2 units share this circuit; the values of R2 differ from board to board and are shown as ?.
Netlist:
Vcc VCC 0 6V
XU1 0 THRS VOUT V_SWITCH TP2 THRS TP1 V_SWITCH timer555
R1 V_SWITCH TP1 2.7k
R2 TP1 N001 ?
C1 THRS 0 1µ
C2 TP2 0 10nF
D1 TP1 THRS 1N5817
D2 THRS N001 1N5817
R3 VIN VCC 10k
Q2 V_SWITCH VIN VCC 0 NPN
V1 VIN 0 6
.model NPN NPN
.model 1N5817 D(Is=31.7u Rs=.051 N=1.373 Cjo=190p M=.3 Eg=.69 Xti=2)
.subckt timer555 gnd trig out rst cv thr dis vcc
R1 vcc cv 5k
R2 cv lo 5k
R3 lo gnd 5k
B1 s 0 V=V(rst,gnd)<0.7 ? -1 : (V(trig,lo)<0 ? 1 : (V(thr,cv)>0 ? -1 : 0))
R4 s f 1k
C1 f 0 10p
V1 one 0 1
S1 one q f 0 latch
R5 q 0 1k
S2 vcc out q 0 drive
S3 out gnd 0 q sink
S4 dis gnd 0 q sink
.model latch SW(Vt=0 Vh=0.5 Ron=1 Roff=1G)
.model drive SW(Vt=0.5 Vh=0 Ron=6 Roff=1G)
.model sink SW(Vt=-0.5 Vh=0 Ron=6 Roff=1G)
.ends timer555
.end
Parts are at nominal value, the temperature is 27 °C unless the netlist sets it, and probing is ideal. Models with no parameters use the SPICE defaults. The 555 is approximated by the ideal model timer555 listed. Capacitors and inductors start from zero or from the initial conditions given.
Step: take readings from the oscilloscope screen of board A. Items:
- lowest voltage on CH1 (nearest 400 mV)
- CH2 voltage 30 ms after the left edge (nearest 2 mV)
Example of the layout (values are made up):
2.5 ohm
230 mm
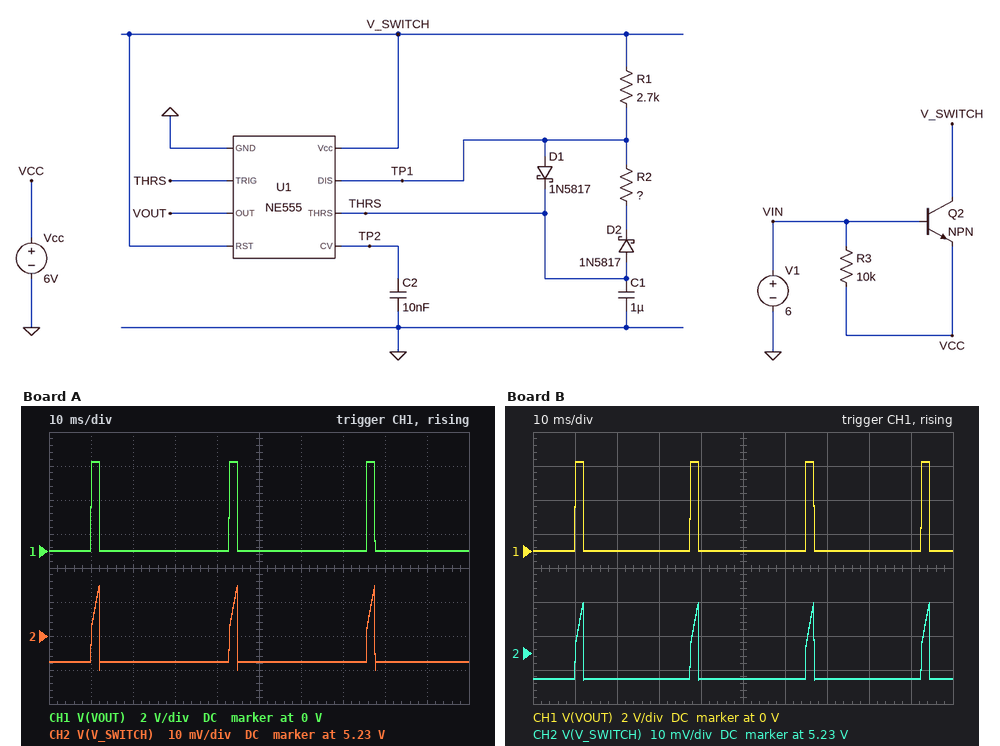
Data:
0 V
5.222 V
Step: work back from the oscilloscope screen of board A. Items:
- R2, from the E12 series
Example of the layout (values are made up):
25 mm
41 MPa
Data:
100 kΩ
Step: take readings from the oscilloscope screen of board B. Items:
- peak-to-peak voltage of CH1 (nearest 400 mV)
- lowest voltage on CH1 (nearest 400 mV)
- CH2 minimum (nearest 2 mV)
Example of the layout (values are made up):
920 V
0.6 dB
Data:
5.2 V
0 V
5.222 V
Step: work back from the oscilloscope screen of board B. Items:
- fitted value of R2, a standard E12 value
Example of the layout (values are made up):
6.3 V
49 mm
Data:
68 kΩ
